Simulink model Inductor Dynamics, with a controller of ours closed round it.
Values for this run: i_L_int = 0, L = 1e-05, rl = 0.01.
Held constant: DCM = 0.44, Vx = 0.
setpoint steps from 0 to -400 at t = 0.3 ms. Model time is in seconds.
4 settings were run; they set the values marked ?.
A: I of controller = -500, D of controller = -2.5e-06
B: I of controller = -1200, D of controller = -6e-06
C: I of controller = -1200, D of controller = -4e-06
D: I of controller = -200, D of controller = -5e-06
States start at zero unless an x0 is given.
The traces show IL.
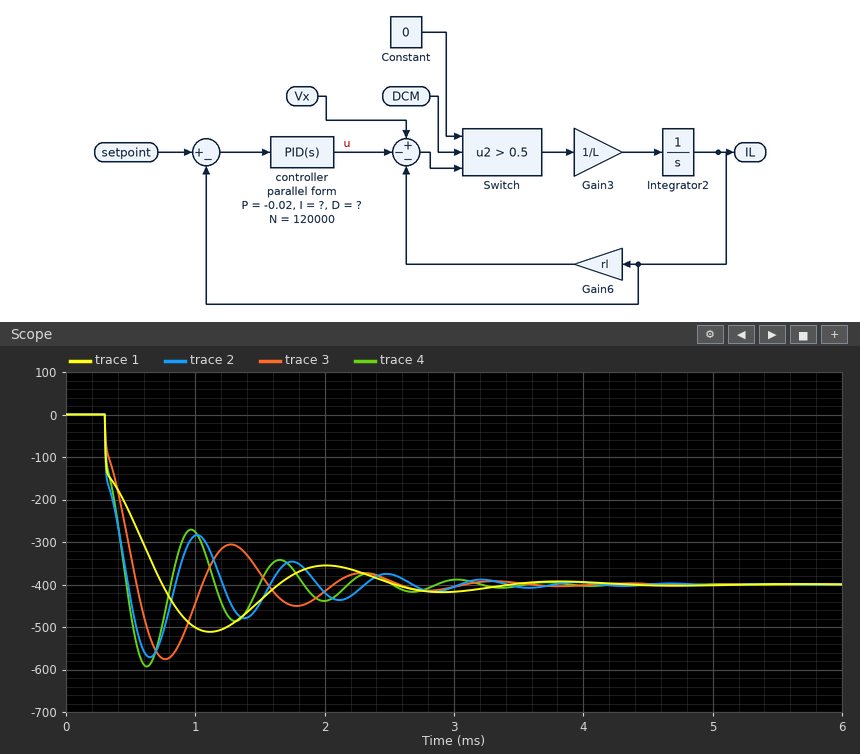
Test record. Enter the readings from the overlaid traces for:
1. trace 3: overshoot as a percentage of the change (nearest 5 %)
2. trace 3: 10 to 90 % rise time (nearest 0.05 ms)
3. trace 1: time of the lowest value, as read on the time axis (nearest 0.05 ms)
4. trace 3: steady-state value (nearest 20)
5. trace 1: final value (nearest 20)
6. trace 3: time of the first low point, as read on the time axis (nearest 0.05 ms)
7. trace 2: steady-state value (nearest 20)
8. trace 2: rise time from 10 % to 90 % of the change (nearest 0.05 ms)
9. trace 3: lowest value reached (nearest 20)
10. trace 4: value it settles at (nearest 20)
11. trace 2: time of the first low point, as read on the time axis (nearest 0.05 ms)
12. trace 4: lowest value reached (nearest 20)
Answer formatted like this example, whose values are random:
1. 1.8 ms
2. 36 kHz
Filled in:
1. 45 %
2. 0.20 ms
3. 1.10 ms
4. -400
5. -400
6. 0.75 ms
7. -400
8. 0.15 ms
9. -580
10. -400
11. 0.65 ms
12. -600
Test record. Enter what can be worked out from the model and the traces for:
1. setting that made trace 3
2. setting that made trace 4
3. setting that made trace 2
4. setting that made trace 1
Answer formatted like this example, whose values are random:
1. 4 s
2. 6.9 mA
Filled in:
1. A
2. C
3. B
4. D
